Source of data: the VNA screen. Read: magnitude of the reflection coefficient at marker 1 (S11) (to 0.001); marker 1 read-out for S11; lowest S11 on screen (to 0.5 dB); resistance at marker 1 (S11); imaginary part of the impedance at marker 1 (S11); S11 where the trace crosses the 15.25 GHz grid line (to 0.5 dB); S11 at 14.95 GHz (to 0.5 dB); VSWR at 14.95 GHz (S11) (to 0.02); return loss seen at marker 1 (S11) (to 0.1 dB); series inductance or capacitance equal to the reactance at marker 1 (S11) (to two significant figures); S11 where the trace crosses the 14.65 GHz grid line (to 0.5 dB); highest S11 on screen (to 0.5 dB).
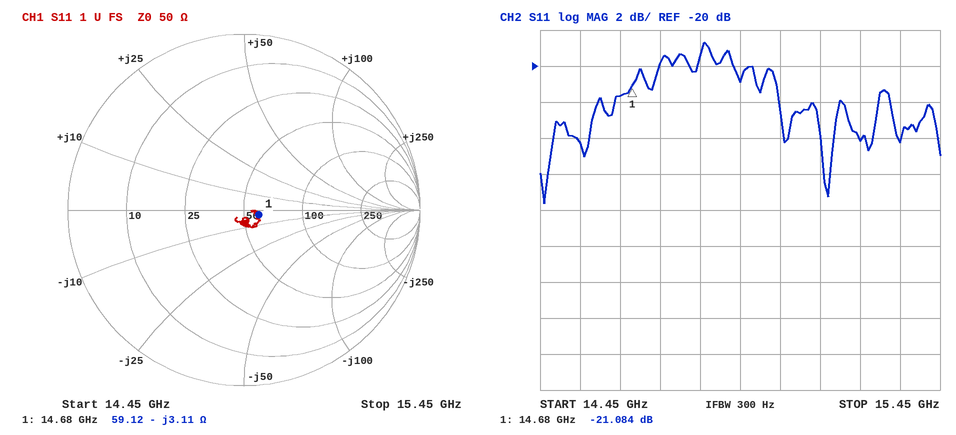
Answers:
0.088
-21.084 dB
-27.5 dB
59.12 Ω
-3.11 Ω
-24.0 dB
-21.0 dB
1.20
21.1 dB
3.5 pF
-21.5 dB
-18.5 dB
